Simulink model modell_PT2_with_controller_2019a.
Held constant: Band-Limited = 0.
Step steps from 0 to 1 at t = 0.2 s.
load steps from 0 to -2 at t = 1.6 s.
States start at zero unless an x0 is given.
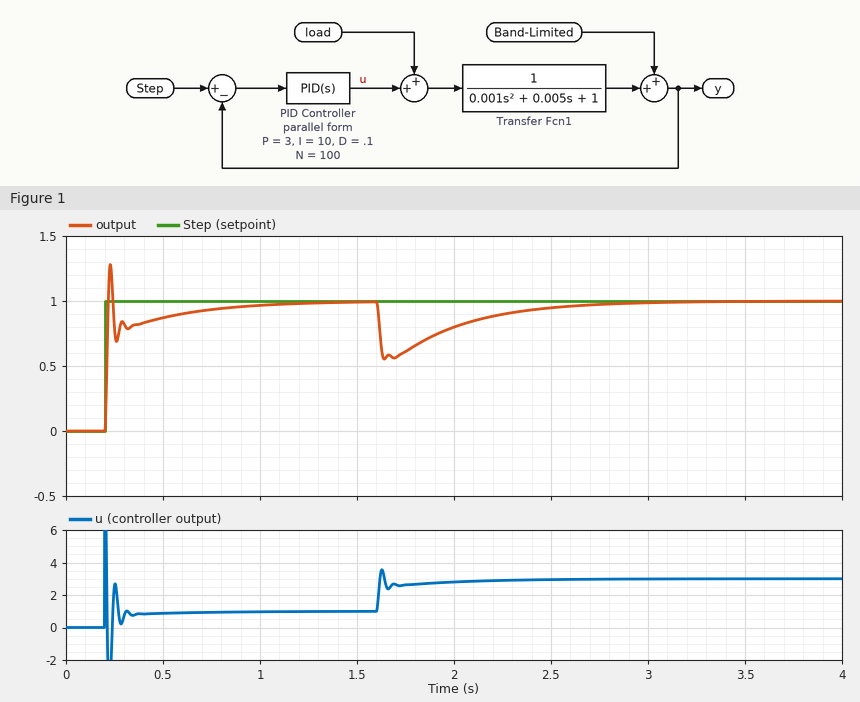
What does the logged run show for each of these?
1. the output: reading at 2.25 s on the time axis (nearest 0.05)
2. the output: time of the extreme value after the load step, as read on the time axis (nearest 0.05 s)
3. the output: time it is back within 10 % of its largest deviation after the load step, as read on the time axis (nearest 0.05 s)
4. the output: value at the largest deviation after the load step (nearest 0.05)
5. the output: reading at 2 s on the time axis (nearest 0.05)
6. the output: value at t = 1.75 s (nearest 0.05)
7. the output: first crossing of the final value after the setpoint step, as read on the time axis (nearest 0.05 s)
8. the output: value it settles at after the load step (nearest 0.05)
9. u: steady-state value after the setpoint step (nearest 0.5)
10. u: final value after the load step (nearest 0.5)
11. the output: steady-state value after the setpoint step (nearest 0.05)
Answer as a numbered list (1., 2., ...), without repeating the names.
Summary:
1. 0.90
2. 1.65 s
3. 2.55 s
4. 0.55
5. 0.80
6. 0.60
7. 0.20 s
8. 1.00
9. 1.0
10. 3.0
11. 1.00
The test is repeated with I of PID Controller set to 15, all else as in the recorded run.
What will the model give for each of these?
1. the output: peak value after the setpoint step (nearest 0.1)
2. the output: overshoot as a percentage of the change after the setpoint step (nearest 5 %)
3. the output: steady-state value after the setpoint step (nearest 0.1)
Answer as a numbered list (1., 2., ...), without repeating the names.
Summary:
1. 1.3
2. 30 %
3. 1.0
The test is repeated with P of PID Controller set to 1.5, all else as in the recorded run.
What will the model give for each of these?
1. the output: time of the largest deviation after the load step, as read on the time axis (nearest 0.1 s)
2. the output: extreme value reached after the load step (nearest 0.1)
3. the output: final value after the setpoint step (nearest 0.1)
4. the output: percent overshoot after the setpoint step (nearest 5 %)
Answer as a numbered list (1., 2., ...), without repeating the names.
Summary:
1. 1.7 s
2. 0.4
3. 1.0
4. 15 %
